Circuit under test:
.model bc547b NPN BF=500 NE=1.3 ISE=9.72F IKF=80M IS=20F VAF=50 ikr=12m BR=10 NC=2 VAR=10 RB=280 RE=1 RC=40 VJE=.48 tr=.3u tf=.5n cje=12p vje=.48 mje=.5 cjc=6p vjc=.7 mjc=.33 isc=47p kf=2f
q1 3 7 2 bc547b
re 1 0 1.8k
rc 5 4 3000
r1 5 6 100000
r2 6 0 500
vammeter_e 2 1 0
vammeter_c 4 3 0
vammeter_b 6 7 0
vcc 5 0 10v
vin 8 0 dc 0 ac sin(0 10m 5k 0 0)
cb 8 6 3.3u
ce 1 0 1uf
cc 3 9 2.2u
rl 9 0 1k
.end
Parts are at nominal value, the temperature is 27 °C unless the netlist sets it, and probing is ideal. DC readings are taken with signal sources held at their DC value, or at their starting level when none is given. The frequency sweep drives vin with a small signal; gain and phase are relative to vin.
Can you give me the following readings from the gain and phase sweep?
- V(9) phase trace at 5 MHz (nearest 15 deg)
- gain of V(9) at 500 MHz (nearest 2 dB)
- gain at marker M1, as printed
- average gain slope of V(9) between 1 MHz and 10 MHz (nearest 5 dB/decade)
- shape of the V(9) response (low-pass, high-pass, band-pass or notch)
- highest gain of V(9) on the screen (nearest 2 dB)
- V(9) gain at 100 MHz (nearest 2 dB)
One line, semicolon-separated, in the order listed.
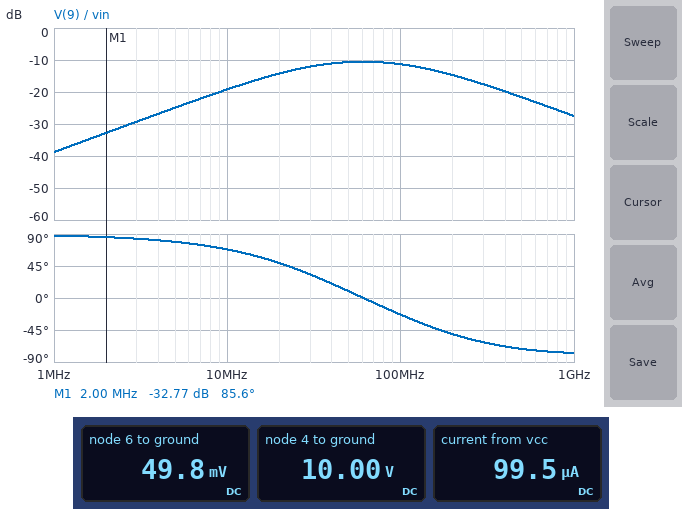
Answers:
75 deg; -22 dB; -32.77 dB; 20 dB/decade; band-pass; -10 dB; -12 dB
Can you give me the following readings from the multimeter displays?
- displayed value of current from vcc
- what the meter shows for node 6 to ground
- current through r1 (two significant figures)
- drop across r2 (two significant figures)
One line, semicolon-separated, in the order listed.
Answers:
99.5 µA; 49.8 mV; 100 µA; 50 mV
